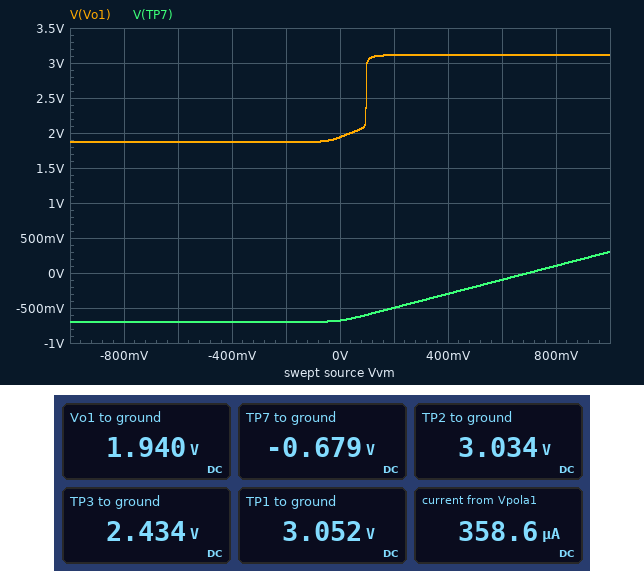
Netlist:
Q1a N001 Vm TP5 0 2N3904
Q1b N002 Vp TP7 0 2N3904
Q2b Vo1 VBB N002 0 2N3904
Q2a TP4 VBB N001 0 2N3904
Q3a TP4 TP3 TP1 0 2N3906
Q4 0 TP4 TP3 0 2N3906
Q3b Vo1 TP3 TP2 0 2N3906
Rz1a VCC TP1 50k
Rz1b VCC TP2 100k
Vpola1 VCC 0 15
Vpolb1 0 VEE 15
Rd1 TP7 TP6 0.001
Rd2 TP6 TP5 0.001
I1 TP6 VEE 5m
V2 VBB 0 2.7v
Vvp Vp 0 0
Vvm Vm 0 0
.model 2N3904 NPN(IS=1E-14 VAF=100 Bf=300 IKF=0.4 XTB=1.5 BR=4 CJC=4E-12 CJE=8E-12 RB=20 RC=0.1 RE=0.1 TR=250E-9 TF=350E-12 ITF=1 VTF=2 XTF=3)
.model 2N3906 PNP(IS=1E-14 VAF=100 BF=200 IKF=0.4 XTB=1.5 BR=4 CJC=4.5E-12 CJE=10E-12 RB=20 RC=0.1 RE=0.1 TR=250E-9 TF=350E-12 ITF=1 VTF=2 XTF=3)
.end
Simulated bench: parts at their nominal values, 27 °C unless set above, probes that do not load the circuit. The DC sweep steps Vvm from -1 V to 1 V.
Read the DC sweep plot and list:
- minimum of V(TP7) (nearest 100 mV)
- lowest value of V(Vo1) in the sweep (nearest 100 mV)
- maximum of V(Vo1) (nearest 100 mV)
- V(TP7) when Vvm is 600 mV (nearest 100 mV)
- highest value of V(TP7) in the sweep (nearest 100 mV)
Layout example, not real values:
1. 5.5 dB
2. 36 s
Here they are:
1. -700 mV
2. 1.9 V
3. 3.1 V
4. -100 mV
5. 300 mV
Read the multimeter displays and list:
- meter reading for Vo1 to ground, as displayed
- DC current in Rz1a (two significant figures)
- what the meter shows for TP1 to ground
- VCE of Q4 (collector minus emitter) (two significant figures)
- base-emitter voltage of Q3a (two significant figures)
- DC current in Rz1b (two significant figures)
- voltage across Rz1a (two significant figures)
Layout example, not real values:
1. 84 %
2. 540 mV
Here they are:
1. 1.940 V
2. 240 µA
3. 3.052 V
4. -2.4 V
5. -620 mV
6. 120 µA
7. 12 V
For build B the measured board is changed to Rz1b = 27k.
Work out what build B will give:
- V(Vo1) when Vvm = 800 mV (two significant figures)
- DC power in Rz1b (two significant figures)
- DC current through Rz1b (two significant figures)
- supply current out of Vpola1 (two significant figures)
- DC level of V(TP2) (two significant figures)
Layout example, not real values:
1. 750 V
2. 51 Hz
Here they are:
1. 3.2 V
2. 5.3 mW
3. 440 µA
4. 680 µA
5. 3.1 V
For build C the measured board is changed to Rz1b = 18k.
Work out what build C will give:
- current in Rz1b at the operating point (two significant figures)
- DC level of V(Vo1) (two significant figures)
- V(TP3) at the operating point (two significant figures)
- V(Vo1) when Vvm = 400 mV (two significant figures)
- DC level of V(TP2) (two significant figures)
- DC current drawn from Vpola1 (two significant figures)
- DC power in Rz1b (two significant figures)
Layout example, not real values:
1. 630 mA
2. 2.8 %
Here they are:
1. 660 µA
2. 2.0 V
3. 2.5 V
4. 3.2 V
5. 3.1 V
6. 900 µA
7. 7.9 mW
